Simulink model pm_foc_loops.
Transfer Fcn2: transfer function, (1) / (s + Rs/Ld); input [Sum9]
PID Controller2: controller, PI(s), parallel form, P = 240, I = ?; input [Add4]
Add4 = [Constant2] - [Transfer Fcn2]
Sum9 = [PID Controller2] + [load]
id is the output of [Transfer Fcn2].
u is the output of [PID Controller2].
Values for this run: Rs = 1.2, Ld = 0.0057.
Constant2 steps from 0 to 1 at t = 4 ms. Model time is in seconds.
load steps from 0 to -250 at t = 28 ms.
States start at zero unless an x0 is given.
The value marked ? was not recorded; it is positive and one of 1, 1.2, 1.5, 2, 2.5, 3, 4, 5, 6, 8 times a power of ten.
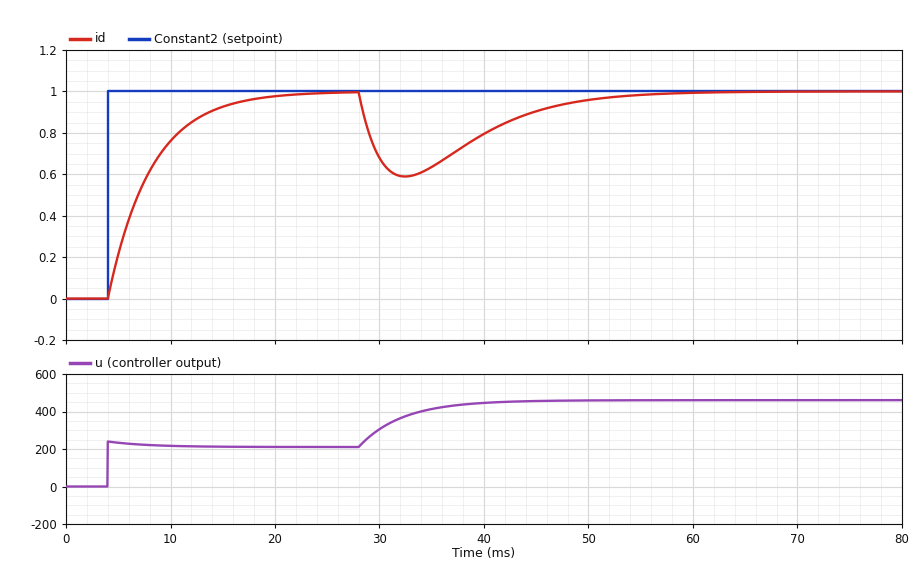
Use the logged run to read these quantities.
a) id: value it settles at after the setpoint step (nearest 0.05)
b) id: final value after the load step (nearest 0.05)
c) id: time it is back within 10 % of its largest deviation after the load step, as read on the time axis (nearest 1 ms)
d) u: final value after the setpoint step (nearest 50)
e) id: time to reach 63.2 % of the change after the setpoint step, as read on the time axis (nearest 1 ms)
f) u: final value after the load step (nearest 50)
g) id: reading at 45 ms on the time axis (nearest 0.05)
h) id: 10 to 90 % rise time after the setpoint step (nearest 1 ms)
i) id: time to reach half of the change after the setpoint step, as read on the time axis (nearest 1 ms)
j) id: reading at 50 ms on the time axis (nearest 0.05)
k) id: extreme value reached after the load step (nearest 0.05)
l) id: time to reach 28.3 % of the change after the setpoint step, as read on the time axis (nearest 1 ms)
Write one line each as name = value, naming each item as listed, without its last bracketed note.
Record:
id: value it settles at after the setpoint step = 1.00
id: final value after the load step = 1.00
id: time it is back within 10 % of its largest deviation after the load step, as read on the time axis = 50 ms
u: final value after the setpoint step = 200
id: time to reach 63.2 % of the change after the setpoint step, as read on the time axis = 8 ms
u: final value after the load step = 450
id: reading at 45 ms on the time axis = 0.90
id: 10 to 90 % rise time after the setpoint step = 9 ms
id: time to reach half of the change after the setpoint step, as read on the time axis = 7 ms
id: reading at 50 ms on the time axis = 0.95
id: extreme value reached after the load step = 0.60
id: time to reach 28.3 % of the change after the setpoint step, as read on the time axis = 5 ms
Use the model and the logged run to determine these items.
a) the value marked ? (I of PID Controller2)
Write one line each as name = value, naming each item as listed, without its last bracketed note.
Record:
the value marked ? = 50000
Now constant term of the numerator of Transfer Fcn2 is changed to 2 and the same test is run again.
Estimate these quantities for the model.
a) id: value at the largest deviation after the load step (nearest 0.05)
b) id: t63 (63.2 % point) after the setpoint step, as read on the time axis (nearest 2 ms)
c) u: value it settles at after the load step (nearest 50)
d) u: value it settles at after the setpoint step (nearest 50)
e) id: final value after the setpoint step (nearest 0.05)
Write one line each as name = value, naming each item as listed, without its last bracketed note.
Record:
id: value at the largest deviation after the load step = 0.45
id: t63 (63.2 % point) after the setpoint step, as read on the time axis = 6 ms
u: value it settles at after the load step = 350
u: value it settles at after the setpoint step = 100
id: final value after the setpoint step = 1.00
